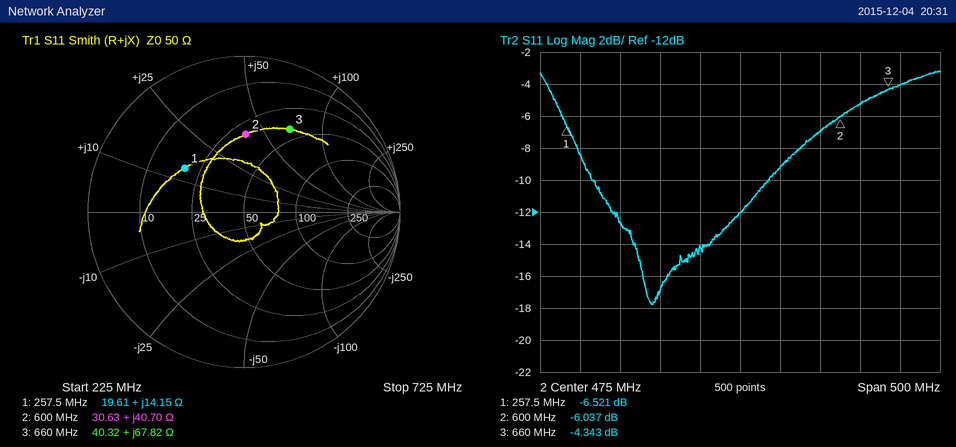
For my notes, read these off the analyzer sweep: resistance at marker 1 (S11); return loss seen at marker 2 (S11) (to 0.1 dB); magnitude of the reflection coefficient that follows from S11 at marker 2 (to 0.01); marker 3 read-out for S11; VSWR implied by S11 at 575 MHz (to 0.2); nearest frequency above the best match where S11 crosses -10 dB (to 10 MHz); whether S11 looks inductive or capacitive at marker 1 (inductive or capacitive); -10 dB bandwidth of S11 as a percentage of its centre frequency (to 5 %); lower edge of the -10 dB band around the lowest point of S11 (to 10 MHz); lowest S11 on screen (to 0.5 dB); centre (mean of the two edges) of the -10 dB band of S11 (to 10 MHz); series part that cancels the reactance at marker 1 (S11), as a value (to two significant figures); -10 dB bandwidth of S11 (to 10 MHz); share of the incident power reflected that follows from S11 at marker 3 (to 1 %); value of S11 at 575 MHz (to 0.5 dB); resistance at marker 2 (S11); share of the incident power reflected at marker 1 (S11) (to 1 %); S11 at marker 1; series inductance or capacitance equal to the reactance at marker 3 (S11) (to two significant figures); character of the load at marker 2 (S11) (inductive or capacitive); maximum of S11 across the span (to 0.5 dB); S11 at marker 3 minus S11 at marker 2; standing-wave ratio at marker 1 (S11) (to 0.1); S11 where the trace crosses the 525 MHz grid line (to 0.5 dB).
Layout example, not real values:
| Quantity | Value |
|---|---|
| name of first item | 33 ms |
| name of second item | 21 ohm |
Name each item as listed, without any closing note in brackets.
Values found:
| Quantity | Value |
|---|---|
| resistance at marker 1 | 19.61 Ω |
| return loss seen at marker 2 (S11) | 6.0 dB |
| magnitude of the reflection coefficient that follows from S11 at marker 2 | 0.50 |
| marker 3 read-out for S11 | -4.343 dB |
| VSWR implied by S11 at 575 MHz | 2.6 |
| nearest frequency above the best match where S11 crosses -10 dB | 510 MHz |
| whether S11 looks inductive or capacitive at marker 1 | inductive |
| -10 dB bandwidth of S11 as a percentage of its centre frequency | 55 % |
| lower edge of the -10 dB band around the lowest point of S11 | 290 MHz |
| lowest S11 on screen | -18.0 dB |
| centre (mean of the two edges) of the -10 dB band of S11 | 400 MHz |
| series part that cancels the reactance at marker 1 (S11), as a value | 44 pF |
| -10 dB bandwidth of S11 | 220 MHz |
| share of the incident power reflected that follows from S11 at marker 3 | 37 % |
| value of S11 at 575 MHz | -7.0 dB |
| resistance at marker 2 | 30.63 Ω |
| share of the incident power reflected at marker 1 (S11) | 22 % |
| S11 at marker 1 | -6.521 dB |
| series inductance or capacitance equal to the reactance at marker 3 (S11) | 16 nH |
| character of the load at marker 2 (S11) | inductive |
| maximum of S11 across the span | -3.0 dB |
| S11 at marker 3 minus S11 at marker 2 | 1.694 dB |
| standing-wave ratio at marker 1 (S11) | 2.8 |
| S11 where the trace crosses the 525 MHz grid line | -9.0 dB |
